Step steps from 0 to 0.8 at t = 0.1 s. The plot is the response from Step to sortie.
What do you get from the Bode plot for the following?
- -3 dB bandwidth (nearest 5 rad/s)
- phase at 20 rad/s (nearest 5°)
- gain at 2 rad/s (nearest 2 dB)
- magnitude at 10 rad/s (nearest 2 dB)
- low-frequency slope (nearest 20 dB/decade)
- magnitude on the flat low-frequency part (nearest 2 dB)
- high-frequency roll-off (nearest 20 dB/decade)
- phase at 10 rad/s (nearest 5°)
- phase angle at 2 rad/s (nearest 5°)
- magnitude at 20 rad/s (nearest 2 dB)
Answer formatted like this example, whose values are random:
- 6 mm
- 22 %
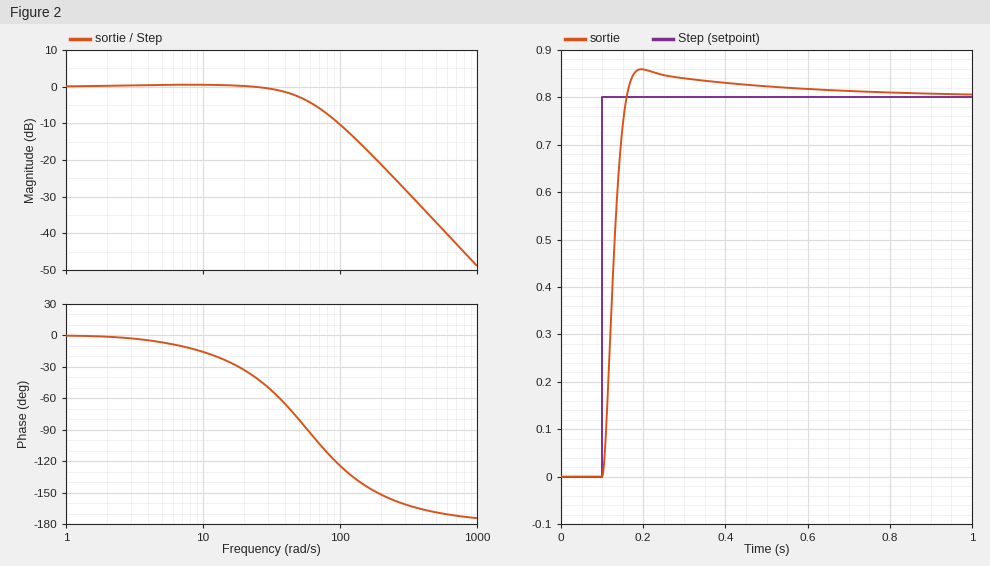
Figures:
- 50 rad/s
- -35°
- 0 dB
- 0 dB
- 0 dB/decade
- 0 dB
- -40 dB/decade
- -15°
- 0°
- 0 dB
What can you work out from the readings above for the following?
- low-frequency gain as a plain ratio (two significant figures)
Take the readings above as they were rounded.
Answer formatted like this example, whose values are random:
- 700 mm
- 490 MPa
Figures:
- 1.0
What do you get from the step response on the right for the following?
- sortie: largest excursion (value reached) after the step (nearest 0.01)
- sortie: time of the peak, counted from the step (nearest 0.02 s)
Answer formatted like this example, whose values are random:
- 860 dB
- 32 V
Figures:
- 0.86
- 0.10 s
